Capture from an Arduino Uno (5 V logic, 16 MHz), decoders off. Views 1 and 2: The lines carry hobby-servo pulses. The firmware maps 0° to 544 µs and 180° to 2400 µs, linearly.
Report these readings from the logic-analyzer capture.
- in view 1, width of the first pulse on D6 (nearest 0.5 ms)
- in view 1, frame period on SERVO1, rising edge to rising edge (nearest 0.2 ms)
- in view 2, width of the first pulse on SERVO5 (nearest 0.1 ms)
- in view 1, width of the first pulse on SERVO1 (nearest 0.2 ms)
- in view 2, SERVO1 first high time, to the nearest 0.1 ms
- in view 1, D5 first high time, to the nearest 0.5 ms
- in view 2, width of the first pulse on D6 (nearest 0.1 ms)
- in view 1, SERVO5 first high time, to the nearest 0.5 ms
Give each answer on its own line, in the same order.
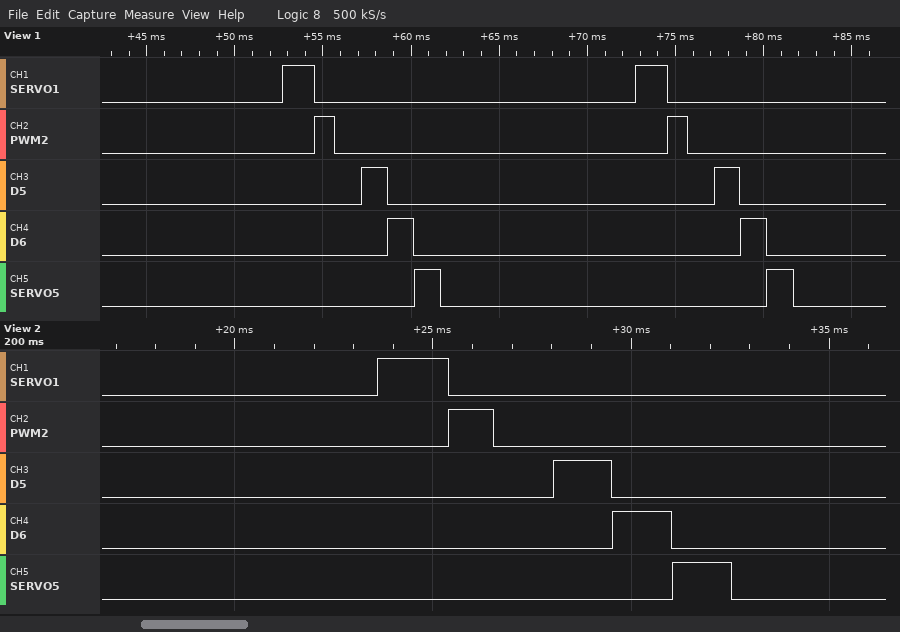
1.5 ms
20.0 ms
1.5 ms
1.8 ms
1.8 ms
1.5 ms
1.5 ms
1.5 ms
